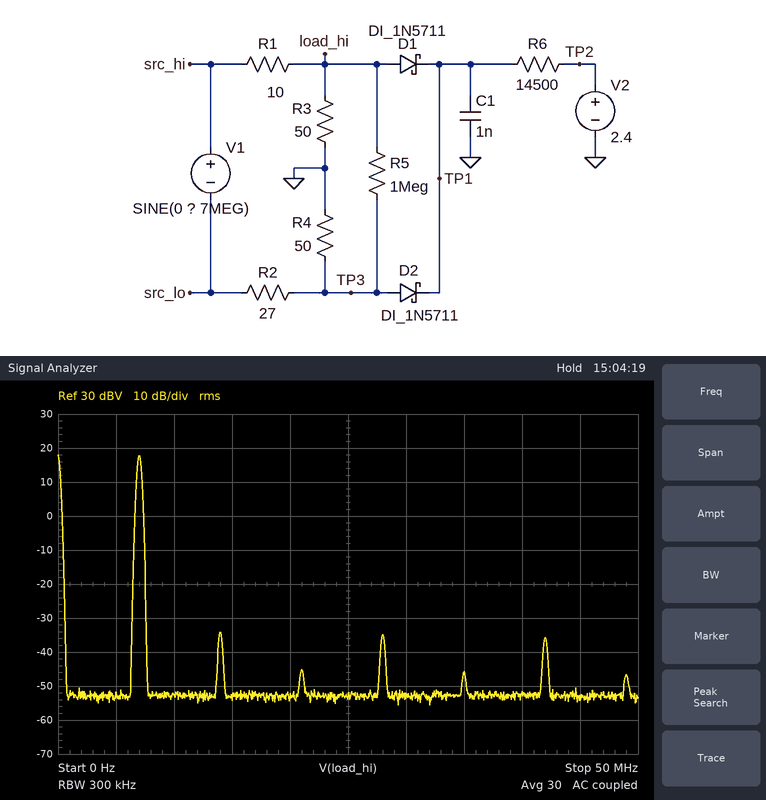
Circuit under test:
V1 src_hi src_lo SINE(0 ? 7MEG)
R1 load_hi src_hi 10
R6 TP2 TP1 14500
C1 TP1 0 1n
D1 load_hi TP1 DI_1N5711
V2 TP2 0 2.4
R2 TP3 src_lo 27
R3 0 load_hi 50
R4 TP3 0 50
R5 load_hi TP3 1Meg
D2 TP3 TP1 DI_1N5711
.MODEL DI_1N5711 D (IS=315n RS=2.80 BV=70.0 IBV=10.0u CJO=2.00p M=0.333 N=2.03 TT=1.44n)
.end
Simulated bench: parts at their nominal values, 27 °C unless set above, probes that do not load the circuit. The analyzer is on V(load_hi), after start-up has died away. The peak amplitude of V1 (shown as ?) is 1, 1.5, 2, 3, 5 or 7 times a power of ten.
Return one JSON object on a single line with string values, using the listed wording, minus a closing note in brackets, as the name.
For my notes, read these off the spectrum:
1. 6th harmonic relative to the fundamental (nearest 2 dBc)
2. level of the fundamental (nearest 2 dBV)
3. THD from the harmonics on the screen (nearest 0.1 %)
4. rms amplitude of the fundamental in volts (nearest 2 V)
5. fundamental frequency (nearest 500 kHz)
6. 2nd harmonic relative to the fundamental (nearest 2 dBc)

{"6th harmonic relative to the fundamental": "-54 dBc", "level of the fundamental": "18 dBV", "THD from the harmonics on the screen": "0.4 %", "rms amplitude of the fundamental in volts": "8 V", "fundamental frequency": "7.0 MHz", "2nd harmonic relative to the fundamental": "-52 dBc"}
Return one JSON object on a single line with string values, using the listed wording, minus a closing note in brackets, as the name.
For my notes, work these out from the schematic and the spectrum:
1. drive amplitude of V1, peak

{"drive amplitude of V1, peak": "30 V"}
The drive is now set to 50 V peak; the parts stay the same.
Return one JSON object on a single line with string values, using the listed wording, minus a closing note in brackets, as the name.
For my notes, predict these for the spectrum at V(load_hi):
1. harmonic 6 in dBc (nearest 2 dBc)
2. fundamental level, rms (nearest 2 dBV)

{"harmonic 6 in dBc": "-52 dBc", "fundamental level, rms": "22 dBV"}
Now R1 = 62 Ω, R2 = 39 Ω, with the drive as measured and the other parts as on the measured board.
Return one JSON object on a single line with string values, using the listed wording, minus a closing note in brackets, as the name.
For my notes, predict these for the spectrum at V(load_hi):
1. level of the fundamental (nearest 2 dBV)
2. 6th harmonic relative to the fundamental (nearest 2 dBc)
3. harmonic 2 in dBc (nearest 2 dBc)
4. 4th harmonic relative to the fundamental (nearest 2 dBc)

{"level of the fundamental": "14 dBV", "6th harmonic relative to the fundamental": "-56 dBc", "harmonic 2 in dBc": "-54 dBc", "4th harmonic relative to the fundamental": "-54 dBc"}
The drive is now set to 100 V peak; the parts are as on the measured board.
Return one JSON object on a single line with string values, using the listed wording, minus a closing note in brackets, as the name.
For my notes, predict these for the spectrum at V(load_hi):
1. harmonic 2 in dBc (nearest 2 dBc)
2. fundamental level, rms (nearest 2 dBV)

{"harmonic 2 in dBc": "-50 dBc", "fundamental level, rms": "28 dBV"}
